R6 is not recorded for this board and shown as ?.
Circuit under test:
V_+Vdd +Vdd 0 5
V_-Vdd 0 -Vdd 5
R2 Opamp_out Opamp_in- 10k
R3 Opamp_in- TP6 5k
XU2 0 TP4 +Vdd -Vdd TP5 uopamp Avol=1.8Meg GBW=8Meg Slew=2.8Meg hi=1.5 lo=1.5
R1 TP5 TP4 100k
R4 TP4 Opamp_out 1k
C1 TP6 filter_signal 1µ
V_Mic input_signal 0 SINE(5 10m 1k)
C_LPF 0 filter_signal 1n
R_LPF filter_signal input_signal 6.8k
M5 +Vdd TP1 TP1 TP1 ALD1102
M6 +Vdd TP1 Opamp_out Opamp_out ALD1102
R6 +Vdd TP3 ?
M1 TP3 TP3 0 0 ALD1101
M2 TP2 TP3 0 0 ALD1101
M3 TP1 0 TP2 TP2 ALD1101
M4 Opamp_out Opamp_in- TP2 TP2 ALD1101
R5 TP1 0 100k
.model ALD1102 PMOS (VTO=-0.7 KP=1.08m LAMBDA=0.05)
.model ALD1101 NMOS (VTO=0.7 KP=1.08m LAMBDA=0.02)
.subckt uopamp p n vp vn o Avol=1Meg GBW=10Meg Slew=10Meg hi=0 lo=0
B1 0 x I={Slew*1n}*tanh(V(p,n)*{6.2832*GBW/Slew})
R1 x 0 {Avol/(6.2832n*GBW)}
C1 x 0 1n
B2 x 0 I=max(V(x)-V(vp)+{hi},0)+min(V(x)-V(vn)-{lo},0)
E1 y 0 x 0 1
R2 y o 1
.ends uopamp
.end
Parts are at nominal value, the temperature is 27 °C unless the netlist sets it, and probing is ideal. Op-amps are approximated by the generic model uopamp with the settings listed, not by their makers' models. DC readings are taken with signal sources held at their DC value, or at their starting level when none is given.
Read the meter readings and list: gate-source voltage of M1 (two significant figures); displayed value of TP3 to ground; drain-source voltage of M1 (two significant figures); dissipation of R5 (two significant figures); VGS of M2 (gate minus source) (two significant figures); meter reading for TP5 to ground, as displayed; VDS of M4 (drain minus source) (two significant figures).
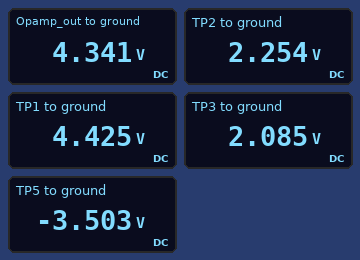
2.1 V
2.085 V
2.1 V
200 µW
2.1 V
-3.503 V
2.1 V
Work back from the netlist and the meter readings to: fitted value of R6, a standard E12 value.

2.7 kΩ
